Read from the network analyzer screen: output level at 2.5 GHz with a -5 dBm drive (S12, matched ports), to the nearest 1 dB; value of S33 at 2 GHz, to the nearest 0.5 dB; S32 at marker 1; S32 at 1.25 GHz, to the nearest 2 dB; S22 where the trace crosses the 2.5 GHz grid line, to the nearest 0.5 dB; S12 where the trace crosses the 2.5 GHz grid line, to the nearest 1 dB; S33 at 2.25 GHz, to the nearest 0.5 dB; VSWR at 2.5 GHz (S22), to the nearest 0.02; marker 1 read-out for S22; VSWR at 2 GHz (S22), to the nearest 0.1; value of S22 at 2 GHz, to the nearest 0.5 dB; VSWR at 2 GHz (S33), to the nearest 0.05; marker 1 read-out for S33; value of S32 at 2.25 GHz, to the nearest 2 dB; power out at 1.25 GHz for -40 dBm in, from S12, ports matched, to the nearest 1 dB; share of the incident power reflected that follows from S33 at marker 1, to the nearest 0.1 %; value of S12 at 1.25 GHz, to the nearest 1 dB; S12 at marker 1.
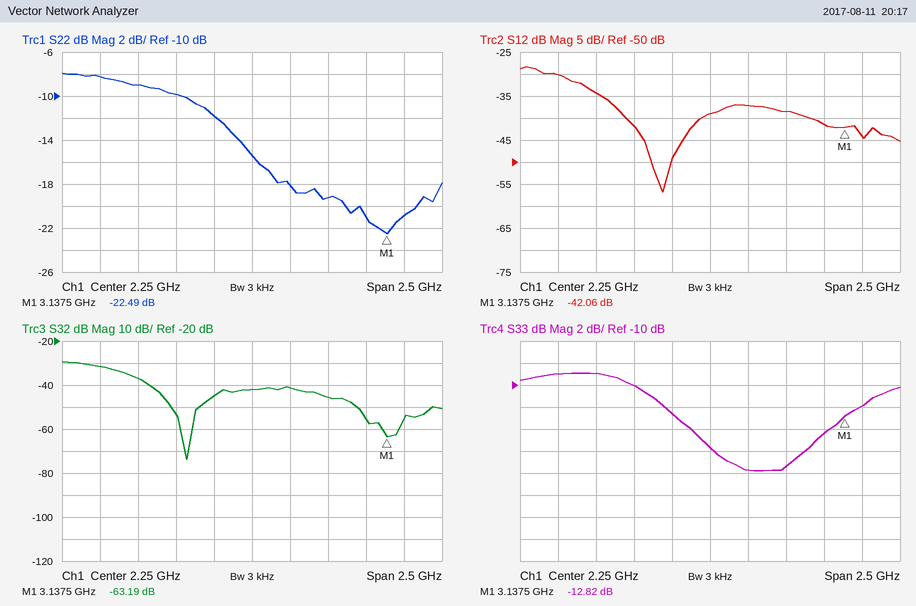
-42 dBm
-12.5 dB
-63.19 dB
-32 dB
-18.0 dB
-37 dB
-15.5 dB
1.28
-22.49 dB
1.7
-12.0 dB
1.60
-12.82 dB
-42 dB
-70 dBm
5.2 %
-30 dB
-42.06 dB
